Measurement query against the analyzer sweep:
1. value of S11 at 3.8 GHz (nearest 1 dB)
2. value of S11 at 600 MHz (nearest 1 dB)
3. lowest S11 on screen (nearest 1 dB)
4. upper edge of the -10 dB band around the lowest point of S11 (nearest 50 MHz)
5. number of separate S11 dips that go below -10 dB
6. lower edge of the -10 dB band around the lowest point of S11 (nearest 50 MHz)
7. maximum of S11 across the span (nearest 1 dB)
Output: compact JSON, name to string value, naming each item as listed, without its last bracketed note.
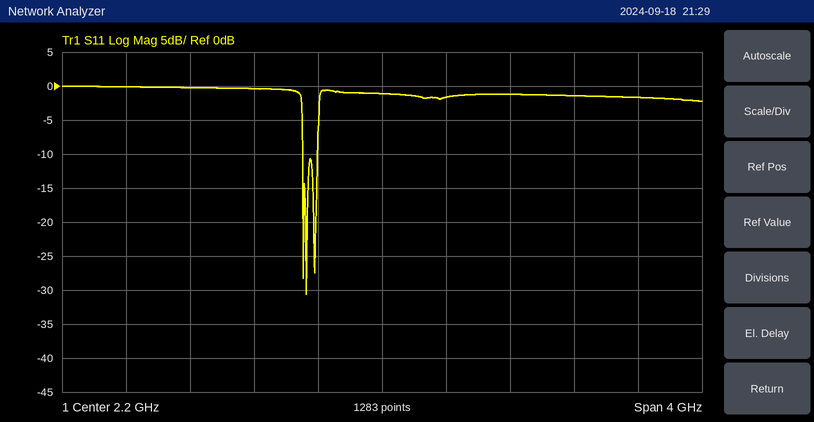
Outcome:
{"value of S11 at 3.8 GHz": "-2 dB", "value of S11 at 600 MHz": "0 dB", "lowest S11 on screen": "-31 dB", "upper edge of the -10 dB band around the lowest point of S11": "1.80 GHz", "number of separate S11 dips that go below -10 dB": "3", "lower edge of the -10 dB band around the lowest point of S11": "1.70 GHz", "maximum of S11 across the span": "0 dB"}
